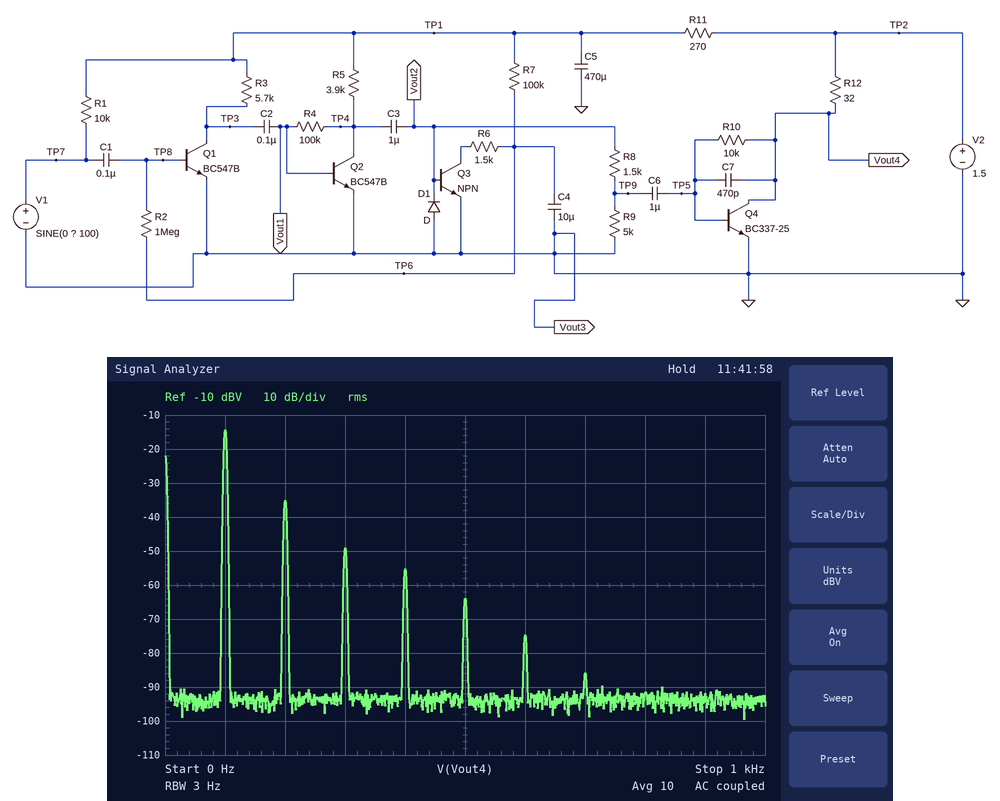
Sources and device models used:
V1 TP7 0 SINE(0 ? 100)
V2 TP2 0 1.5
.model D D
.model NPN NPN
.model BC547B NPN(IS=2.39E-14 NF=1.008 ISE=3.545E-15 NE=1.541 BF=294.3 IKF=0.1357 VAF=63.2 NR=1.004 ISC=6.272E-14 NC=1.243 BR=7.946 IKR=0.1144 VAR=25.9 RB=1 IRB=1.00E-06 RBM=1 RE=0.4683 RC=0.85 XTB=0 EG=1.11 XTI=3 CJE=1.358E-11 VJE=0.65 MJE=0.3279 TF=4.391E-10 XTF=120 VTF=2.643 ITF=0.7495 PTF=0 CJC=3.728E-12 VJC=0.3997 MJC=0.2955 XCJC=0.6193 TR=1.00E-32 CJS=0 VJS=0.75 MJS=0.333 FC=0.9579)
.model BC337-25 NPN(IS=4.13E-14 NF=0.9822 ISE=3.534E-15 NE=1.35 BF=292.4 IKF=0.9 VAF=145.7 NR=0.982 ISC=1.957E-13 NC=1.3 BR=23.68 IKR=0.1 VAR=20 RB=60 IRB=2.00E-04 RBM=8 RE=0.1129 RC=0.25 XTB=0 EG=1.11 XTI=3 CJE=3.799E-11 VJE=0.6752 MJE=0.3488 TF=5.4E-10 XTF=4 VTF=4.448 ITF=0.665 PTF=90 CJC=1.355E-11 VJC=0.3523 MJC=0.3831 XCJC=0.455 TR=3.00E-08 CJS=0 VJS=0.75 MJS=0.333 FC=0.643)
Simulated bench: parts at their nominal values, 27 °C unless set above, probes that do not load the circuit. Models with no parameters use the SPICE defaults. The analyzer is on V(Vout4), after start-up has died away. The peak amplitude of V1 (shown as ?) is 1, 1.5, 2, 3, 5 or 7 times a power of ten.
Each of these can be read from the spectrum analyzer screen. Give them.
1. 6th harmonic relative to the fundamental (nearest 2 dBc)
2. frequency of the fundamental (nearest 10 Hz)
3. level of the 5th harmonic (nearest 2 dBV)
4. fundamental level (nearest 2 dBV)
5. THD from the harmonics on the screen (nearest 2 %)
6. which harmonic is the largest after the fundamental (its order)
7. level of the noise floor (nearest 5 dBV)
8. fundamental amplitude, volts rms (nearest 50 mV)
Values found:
-60 dBc
100 Hz
-64 dBV
-14 dBV
10 %
2
-95 dBV
200 mV
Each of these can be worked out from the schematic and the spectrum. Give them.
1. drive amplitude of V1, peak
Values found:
1.5 mV
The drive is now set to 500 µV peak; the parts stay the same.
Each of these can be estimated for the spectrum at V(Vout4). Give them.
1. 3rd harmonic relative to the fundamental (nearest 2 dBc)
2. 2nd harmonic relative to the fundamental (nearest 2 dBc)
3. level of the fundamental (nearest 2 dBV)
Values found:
-52 dBc
-30 dBc
-24 dBV
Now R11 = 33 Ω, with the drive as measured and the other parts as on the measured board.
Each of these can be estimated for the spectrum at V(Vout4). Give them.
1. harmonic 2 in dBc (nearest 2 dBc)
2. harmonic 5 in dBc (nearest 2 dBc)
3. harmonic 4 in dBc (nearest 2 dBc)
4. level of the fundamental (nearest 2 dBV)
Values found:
-22 dBc
-48 dBc
-38 dBc
-14 dBV
